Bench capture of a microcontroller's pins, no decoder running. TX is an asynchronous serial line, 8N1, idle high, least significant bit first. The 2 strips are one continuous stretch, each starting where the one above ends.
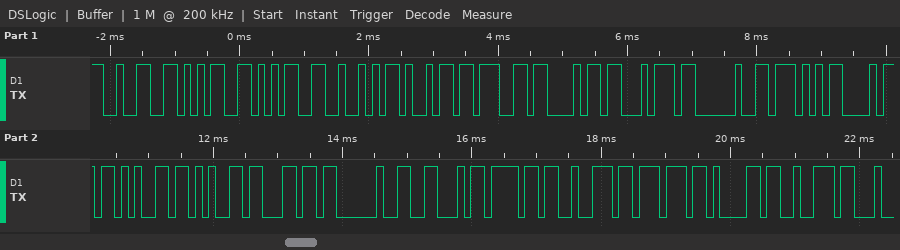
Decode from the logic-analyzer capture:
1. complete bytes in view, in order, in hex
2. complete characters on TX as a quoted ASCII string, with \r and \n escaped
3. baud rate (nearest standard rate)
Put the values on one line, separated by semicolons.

32 35 35 52 69 67 68 74 20 57 68 65 65 6C 20 46 6F 72 77 61 72; "255Right Wheel Forwar"; 9600 baud
